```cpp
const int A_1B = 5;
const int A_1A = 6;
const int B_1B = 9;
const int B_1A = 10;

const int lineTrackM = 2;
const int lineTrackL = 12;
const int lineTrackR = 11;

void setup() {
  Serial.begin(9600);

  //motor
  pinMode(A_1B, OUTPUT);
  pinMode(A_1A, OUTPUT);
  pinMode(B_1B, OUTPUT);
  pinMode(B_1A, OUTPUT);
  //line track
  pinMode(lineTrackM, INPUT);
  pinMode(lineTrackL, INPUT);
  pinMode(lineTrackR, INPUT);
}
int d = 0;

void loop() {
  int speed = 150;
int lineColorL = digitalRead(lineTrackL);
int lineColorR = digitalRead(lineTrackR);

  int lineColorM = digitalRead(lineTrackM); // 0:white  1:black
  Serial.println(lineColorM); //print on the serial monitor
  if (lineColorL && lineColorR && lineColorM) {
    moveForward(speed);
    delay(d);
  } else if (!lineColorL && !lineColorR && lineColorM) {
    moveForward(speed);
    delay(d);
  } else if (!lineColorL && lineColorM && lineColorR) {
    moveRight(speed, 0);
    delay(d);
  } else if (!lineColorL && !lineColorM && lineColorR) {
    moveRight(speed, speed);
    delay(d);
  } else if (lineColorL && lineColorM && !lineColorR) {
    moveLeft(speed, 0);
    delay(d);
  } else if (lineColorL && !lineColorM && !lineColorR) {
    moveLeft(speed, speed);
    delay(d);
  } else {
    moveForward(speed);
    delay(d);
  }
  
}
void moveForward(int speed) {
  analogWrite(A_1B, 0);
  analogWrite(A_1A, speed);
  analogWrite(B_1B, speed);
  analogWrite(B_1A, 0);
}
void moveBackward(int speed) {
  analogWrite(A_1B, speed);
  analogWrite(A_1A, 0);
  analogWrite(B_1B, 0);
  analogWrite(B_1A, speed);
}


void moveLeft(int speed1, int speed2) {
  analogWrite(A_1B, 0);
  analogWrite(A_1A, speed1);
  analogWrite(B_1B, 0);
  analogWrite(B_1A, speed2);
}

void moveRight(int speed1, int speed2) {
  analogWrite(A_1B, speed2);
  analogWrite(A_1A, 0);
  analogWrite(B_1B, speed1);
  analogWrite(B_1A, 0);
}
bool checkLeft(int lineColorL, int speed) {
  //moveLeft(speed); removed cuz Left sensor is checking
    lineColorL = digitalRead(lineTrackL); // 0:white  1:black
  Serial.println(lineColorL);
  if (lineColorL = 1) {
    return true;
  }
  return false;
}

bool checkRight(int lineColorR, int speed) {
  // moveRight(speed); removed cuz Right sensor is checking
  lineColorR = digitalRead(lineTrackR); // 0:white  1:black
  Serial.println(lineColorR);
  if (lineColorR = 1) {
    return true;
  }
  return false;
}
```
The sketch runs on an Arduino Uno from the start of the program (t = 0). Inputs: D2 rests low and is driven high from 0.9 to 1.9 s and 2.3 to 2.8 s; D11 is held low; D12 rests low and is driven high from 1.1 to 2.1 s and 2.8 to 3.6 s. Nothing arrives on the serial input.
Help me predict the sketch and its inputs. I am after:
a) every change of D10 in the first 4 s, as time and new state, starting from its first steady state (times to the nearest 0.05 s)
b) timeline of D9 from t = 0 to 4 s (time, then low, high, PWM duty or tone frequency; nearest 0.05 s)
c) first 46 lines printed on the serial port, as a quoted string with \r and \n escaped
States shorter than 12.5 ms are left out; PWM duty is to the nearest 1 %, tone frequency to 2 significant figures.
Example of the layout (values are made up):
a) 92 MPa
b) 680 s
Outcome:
a) 0 s low; 1.9 s PWM 59 %; 2.1 s low; 2.8 s PWM 59 %; 3.6 s low
b) 0 s PWM 59 %; 1.1 s low; 2.1 s PWM 59 %; 2.8 s low; 3.6 s PWM 59 %
c) "0\r\n0\r\n0\r\n0\r\n0\r\n0\r\n0\r\n0\r\n0\r\n0\r\n0\r\n0\r\n0\r\n0\r\n0\r\n0\r\n0\r\n0\r\n0\r\n0\r\n0\r\n0\r\n0\r\n0\r\n0\r\n0\r\n0\r\n0\r\n0\r\n0\r\n0\r\n0\r\n0\r\n0\r\n0\r\n0\r\n0\r\n0\r\n0\r\n0\r\n0\r\n0\r\n0\r\n0\r\n0\r\n0\r\n"
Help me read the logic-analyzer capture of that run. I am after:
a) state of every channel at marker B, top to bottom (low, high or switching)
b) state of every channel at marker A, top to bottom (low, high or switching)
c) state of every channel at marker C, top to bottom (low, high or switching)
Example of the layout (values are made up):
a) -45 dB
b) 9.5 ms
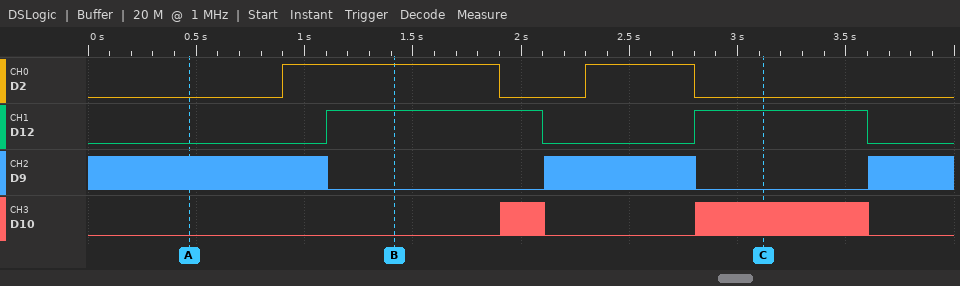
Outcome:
a) D2 high, D12 high, D9 low, D10 low
b) D2 low, D12 low, D9 switching, D10 low
c) D2 low, D12 high, D9 low, D10 switching
